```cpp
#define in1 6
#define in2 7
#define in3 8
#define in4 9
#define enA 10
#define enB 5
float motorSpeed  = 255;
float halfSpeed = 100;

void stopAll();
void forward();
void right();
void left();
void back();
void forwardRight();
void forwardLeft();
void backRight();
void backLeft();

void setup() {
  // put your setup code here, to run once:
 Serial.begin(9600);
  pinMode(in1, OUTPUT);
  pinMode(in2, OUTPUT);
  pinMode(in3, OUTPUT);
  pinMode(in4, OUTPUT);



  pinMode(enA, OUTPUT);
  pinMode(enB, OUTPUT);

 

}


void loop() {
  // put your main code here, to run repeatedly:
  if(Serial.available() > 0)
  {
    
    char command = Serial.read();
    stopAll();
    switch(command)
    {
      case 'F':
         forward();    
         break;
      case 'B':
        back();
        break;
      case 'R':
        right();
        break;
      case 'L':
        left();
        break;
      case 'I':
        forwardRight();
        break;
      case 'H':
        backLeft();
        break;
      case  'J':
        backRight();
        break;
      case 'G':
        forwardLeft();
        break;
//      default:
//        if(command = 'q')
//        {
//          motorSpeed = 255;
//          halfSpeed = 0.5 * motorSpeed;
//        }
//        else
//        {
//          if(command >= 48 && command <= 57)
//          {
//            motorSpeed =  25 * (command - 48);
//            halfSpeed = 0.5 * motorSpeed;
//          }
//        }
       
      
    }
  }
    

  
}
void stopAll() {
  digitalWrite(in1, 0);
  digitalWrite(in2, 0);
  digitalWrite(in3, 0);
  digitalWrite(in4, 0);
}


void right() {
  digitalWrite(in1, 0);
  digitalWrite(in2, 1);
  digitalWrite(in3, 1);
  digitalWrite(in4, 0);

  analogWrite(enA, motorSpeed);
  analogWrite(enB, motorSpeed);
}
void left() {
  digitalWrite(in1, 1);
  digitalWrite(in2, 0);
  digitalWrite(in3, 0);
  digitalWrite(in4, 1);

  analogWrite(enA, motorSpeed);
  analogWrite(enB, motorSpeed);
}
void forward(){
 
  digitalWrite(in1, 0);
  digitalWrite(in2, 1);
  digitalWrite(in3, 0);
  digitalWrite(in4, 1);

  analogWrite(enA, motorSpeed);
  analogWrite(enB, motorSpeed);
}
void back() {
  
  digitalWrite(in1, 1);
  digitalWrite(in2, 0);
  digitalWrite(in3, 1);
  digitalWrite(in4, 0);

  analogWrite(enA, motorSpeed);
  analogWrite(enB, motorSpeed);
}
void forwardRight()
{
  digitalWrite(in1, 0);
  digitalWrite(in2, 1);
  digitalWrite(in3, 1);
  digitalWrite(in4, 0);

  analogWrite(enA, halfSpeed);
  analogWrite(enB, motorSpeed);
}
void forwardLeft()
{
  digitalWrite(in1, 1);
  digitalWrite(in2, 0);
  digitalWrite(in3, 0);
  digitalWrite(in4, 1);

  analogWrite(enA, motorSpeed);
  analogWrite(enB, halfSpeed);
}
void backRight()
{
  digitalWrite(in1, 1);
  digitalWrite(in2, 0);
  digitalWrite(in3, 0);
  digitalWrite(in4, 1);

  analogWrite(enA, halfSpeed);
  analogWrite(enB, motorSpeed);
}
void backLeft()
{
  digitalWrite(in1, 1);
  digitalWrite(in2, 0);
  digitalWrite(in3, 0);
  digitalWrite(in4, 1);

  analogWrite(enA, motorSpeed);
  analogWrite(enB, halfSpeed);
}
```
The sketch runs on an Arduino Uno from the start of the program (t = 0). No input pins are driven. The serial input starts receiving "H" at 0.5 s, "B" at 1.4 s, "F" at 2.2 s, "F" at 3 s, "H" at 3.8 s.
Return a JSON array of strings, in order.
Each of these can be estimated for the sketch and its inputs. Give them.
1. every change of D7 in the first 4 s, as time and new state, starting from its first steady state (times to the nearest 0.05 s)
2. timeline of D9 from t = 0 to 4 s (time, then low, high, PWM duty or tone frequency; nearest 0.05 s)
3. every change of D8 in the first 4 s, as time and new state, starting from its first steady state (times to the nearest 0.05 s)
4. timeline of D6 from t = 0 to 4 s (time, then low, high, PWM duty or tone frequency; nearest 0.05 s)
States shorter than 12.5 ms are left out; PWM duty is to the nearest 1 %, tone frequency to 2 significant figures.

["0 s low; 2.2 s high; 3.8 s low", "0 s low; 0.5 s high; 1.4 s low; 2.2 s high", "0 s low; 1.4 s high; 2.2 s low", "0 s low; 0.5 s high; 2.2 s low; 3.8 s high"]
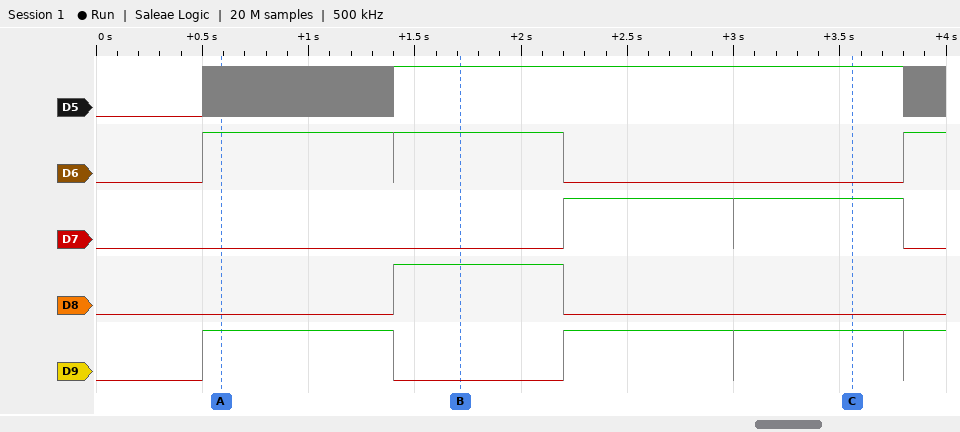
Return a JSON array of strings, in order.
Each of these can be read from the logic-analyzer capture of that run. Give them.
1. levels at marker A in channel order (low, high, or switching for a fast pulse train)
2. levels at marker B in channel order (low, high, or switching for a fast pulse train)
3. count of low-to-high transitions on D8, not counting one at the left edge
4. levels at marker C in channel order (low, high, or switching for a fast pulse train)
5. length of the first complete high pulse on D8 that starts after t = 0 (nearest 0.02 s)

["D5 switching, D6 high, D7 low, D8 low, D9 high", "D5 high, D6 high, D7 low, D8 high, D9 low", "1", "D5 high, D6 low, D7 high, D8 low, D9 high", "0.80 s"]
